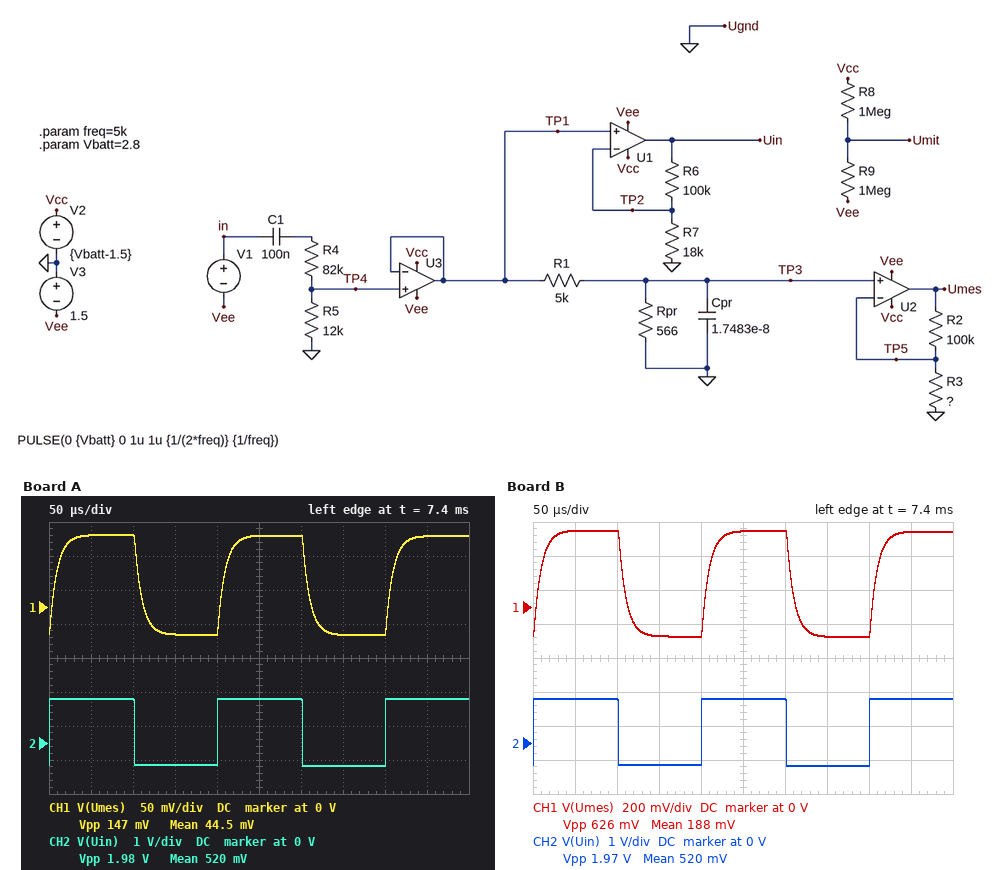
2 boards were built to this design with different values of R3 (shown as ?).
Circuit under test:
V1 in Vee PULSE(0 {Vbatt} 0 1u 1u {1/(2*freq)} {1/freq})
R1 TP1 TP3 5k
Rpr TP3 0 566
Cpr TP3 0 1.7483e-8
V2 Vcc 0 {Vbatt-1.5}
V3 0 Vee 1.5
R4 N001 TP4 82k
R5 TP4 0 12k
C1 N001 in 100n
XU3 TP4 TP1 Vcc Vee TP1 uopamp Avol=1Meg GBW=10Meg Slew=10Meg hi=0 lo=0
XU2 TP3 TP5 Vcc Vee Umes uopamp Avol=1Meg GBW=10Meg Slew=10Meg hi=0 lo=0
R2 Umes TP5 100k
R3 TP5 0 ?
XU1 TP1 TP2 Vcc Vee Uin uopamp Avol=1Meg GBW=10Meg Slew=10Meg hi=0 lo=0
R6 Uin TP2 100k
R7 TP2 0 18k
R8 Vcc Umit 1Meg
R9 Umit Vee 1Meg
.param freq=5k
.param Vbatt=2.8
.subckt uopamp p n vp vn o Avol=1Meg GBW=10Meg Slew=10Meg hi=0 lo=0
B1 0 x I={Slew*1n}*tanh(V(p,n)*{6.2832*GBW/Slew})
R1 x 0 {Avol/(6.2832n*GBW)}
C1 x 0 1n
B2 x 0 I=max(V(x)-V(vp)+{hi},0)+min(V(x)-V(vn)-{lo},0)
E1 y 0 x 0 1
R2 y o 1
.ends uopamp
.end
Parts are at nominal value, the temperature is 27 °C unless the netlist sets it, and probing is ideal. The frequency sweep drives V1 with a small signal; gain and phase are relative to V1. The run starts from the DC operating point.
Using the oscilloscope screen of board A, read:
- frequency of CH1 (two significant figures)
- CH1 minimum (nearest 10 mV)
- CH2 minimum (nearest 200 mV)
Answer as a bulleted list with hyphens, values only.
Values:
- 5.0 kHz
- -40 mV
- -600 mV
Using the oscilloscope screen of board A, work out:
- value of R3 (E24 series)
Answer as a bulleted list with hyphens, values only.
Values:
- 33 kΩ
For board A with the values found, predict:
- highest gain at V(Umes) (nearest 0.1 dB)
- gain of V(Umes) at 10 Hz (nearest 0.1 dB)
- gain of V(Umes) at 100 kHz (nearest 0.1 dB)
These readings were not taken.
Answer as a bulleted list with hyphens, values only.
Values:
- -25.6 dB
- -31.5 dB
- -40.7 dB
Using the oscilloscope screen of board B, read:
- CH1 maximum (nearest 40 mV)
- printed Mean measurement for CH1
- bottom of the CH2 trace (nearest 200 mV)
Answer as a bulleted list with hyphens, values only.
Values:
- 440 mV
- 188 mV
- -600 mV
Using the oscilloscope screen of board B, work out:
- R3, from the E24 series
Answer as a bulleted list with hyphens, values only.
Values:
- 6.2 kΩ
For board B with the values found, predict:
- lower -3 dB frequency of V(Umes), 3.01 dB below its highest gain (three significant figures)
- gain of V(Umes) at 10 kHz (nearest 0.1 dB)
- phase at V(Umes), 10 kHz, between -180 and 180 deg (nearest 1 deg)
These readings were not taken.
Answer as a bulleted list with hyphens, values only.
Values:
- 16.9 Hz
- -14.2 dB
- -30 deg
